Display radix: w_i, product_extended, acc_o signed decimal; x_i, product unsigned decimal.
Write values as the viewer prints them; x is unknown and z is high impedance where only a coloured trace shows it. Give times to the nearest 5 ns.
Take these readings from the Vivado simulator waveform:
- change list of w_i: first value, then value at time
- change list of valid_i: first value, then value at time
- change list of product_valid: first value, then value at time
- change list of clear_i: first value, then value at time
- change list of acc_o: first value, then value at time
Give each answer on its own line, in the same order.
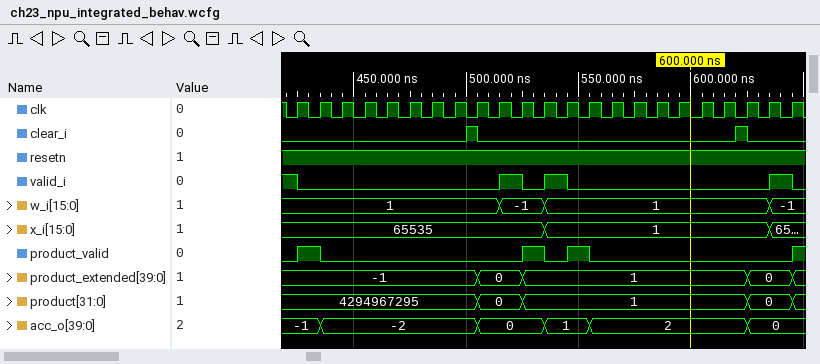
1, -1 at 515 ns, 1 at 535 ns, -1 at 635 ns
1, 0 at 425 ns, 1 at 515 ns, 0 at 525 ns, 1 at 535 ns, 0 at 545 ns, 1 at 635 ns, 0 at 645 ns
0, 1 at 425 ns, 0 at 435 ns, 1 at 525 ns, 0 at 535 ns, 1 at 545 ns, 0 at 555 ns, 1 at 645 ns
0, 1 at 500 ns, 0 at 505 ns, 1 at 620 ns, 0 at 625 ns
-1, -2 at 435 ns, 0 at 505 ns, 1 at 535 ns, 2 at 555 ns, 0 at 625 ns
